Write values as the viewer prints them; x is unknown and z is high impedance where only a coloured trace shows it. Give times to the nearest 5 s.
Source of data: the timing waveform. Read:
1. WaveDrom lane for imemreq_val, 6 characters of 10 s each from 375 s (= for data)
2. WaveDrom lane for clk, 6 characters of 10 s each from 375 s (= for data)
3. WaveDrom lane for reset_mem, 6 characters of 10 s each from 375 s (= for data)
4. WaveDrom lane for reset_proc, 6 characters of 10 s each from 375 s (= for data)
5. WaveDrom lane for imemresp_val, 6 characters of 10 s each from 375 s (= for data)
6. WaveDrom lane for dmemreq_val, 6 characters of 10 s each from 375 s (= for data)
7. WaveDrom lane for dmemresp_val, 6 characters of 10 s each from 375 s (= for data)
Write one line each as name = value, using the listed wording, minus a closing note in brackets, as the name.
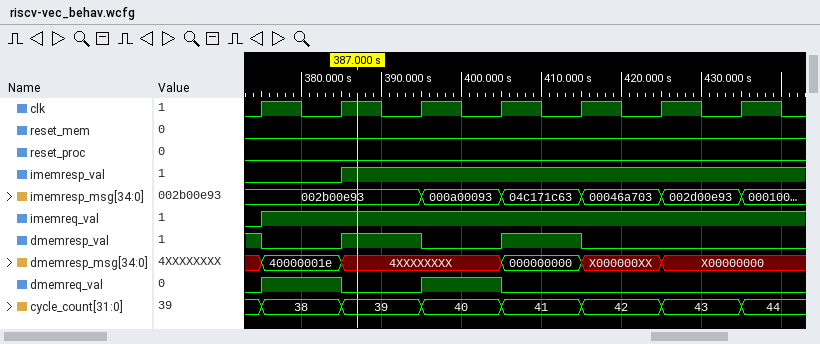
WaveDrom lane for imemreq_val, 6 characters of 10 s each from 375 s = {name: 'imemreq_val', wave: '1.....'}
WaveDrom lane for clk, 6 characters of 10 s each from 375 s = {name: 'clk', wave: 'p.....'}
WaveDrom lane for reset_mem, 6 characters of 10 s each from 375 s = {name: 'reset_mem', wave: '0.....'}
WaveDrom lane for reset_proc, 6 characters of 10 s each from 375 s = {name: 'reset_proc', wave: '0.....'}
WaveDrom lane for imemresp_val, 6 characters of 10 s each from 375 s = {name: 'imemresp_val', wave: '01....'}
WaveDrom lane for dmemreq_val, 6 characters of 10 s each from 375 s = {name: 'dmemreq_val', wave: '1010..'}
WaveDrom lane for dmemresp_val, 6 characters of 10 s each from 375 s = {name: 'dmemresp_val', wave: '01010.'}
